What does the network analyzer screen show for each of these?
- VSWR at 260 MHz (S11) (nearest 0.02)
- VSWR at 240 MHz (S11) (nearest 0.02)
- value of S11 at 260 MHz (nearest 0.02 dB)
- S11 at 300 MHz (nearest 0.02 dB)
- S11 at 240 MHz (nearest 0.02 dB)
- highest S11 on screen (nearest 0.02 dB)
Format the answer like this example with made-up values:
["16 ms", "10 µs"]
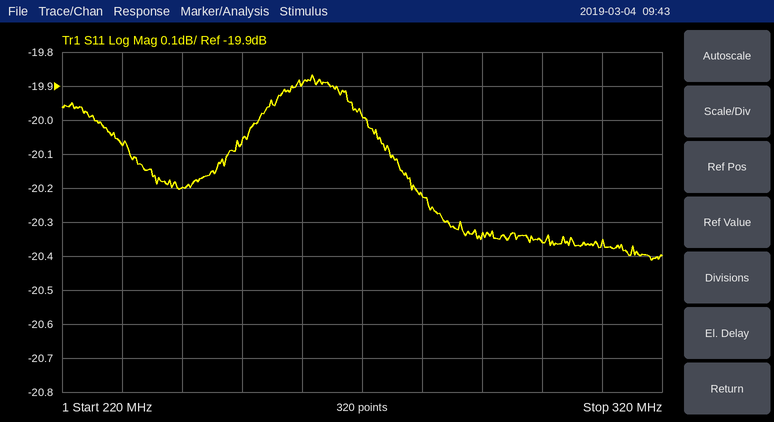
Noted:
["1.22", "1.22", "-19.90 dB", "-20.36 dB", "-20.20 dB", "-19.86 dB"]
